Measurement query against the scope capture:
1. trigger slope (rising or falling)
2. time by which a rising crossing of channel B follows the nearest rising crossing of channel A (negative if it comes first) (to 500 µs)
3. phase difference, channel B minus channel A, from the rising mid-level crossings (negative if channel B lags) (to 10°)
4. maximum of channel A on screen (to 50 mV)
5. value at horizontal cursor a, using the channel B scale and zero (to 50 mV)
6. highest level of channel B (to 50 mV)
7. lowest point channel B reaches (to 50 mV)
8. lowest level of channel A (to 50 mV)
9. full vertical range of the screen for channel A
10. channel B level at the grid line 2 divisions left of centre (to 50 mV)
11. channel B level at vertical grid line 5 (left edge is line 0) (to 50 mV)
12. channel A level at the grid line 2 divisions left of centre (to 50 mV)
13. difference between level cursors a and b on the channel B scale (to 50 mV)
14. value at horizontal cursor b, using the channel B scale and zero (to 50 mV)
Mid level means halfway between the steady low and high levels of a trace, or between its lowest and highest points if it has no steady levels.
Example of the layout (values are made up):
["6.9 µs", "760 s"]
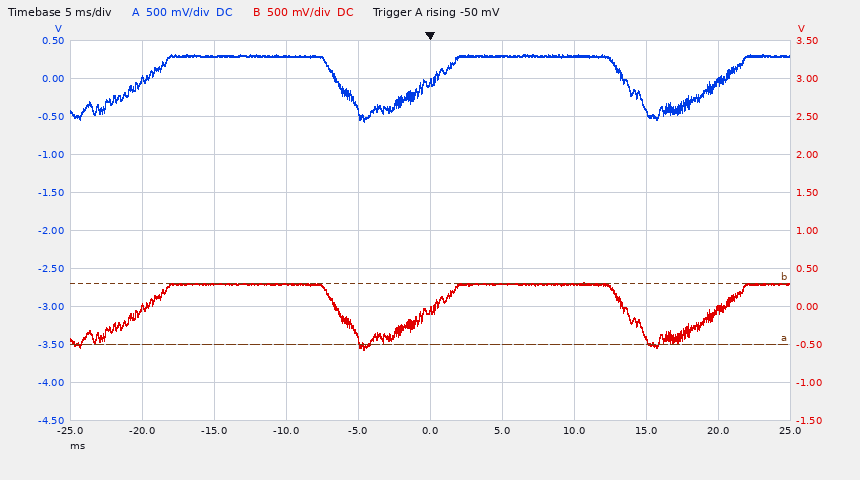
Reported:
["rising", "0.0 ms", "0°", "300 mV", "-500 mV", "300 mV", "-550 mV", "-550 mV", "5 V", "300 mV", "-50 mV", "300 mV", "800 mV", "300 mV"]
